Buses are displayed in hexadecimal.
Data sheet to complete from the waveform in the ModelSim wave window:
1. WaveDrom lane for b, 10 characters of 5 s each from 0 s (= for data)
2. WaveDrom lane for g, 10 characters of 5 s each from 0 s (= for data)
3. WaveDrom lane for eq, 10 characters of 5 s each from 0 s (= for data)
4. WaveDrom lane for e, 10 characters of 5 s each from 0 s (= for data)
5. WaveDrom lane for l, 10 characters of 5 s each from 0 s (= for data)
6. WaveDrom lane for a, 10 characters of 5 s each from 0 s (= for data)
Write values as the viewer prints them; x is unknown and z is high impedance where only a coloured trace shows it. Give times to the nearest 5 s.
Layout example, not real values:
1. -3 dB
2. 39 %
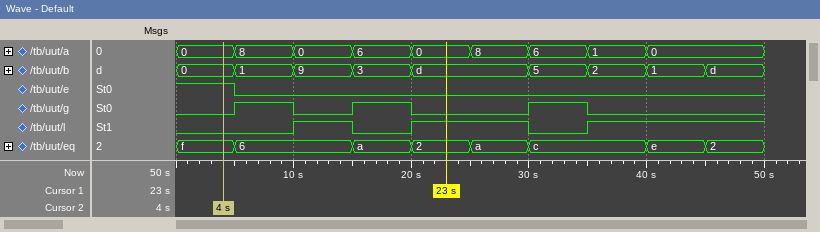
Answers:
1. {name: 'b', wave: '=====.====', data: '0 1 9 3 d 5 2 1 d'}
2. {name: 'g', wave: '01010.10..'}
3. {name: 'eq', wave: '==.====.==', data: 'f 6 a 2 a c e 2'}
4. {name: 'e', wave: '10........'}
5. {name: 'l', wave: '0.101.01..'}
6. {name: 'a', wave: '=========.', data: '0 8 0 6 0 8 6 1 0'}
